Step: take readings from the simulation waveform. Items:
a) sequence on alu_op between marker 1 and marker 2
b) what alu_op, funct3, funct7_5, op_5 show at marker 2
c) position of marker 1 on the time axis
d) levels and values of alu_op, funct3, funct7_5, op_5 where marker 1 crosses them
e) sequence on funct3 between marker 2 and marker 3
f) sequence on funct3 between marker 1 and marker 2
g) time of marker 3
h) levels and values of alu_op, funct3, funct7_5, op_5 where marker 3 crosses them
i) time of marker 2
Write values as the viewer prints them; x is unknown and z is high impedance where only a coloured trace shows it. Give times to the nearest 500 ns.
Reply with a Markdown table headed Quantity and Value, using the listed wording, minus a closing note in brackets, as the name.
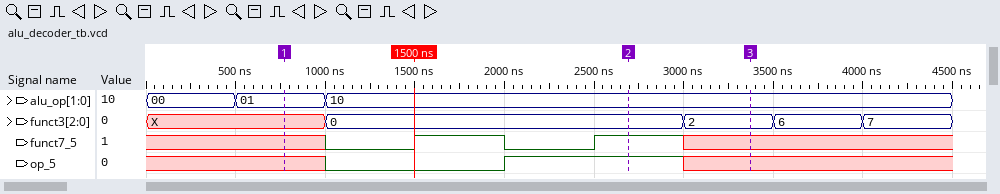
| Quantity | Value |
|---|---|
| sequence on alu_op between marker 1 and marker 2 | 01, 10 |
| what alu_op, funct3, funct7_5, op_5 show at marker 2 | alu_op=10, funct3=0, funct7_5=1, op_5=1 |
| position of marker 1 on the time axis | 1000 ns |
| levels and values of alu_op, funct3, funct7_5, op_5 where marker 1 crosses them | alu_op=01, funct3=X, funct7_5=x, op_5=x |
| sequence on funct3 between marker 2 and marker 3 | 0, 2 |
| sequence on funct3 between marker 1 and marker 2 | X, 0 |
| time of marker 3 | 3500 ns |
| levels and values of alu_op, funct3, funct7_5, op_5 where marker 3 crosses them | alu_op=10, funct3=2, funct7_5=x, op_5=x |
| time of marker 2 | 2500 ns |
